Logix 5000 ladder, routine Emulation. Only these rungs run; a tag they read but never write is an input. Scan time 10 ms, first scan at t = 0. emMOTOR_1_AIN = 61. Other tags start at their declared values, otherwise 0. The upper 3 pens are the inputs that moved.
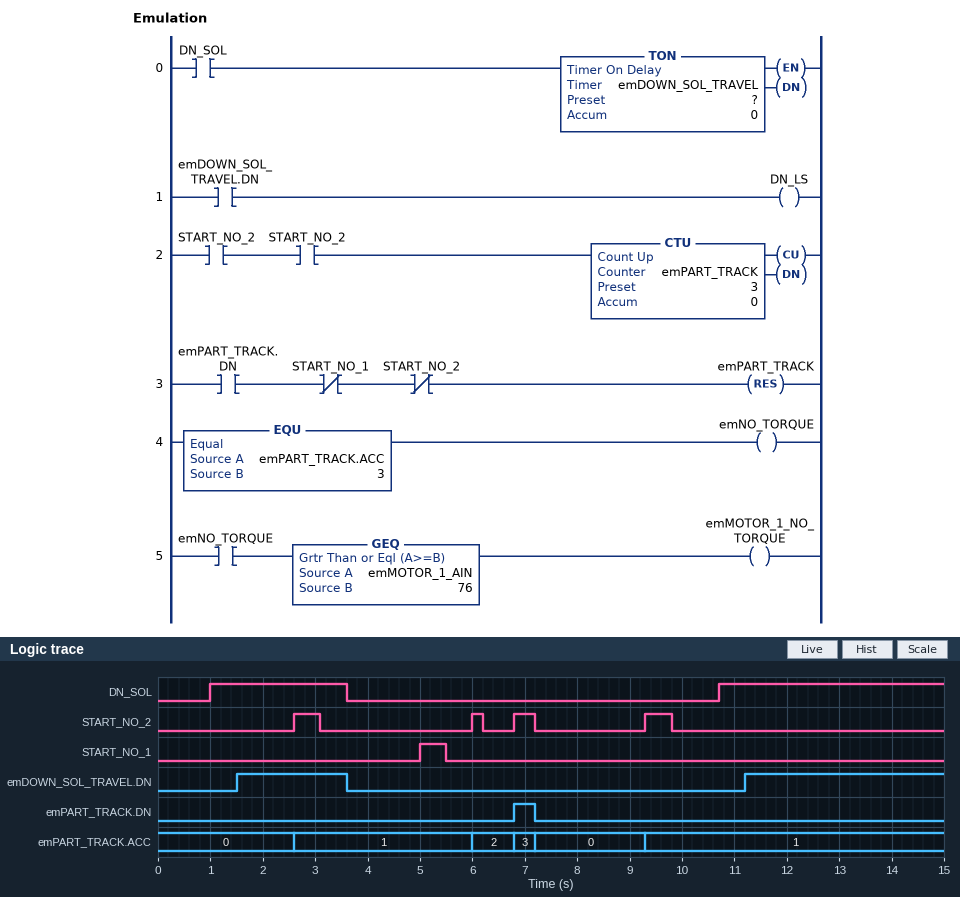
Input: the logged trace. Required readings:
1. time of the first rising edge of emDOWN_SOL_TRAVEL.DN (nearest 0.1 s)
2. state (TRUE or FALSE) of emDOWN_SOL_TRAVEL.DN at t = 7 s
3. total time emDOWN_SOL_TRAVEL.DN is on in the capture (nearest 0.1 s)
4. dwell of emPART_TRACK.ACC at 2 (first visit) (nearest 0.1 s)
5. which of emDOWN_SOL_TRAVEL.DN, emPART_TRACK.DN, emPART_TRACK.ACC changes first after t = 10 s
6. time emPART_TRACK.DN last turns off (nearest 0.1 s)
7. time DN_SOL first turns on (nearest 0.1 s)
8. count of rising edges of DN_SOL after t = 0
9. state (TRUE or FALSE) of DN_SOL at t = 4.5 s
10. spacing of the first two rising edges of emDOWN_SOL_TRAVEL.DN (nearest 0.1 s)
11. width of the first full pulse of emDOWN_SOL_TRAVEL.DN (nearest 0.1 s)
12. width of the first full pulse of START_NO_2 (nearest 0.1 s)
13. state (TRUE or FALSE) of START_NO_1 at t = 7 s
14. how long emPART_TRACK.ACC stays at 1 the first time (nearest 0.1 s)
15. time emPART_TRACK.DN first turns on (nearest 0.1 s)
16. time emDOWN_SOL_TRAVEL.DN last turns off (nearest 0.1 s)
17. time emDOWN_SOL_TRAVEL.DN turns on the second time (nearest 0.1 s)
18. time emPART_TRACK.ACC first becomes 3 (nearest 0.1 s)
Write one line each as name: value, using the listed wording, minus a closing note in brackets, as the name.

time of the first rising edge of emDOWN_SOL_TRAVEL.DN: 1.5 s
state (TRUE or FALSE) of emDOWN_SOL_TRAVEL.DN at t = 7 s: FALSE
total time emDOWN_SOL_TRAVEL.DN is on in the capture: 5.9 s
dwell of emPART_TRACK.ACC at 2 (first visit): 0.8 s
which of emDOWN_SOL_TRAVEL.DN, emPART_TRACK.DN, emPART_TRACK.ACC changes first after t = 10 s: emDOWN_SOL_TRAVEL.DN
time emPART_TRACK.DN last turns off: 7.2 s
time DN_SOL first turns on: 1.0 s
count of rising edges of DN_SOL after t = 0: 2
state (TRUE or FALSE) of DN_SOL at t = 4.5 s: FALSE
spacing of the first two rising edges of emDOWN_SOL_TRAVEL.DN: 9.7 s
width of the first full pulse of emDOWN_SOL_TRAVEL.DN: 2.1 s
width of the first full pulse of START_NO_2: 0.5 s
state (TRUE or FALSE) of START_NO_1 at t = 7 s: FALSE
how long emPART_TRACK.ACC stays at 1 the first time: 3.4 s
time emPART_TRACK.DN first turns on: 6.8 s
time emDOWN_SOL_TRAVEL.DN last turns off: 3.6 s
time emDOWN_SOL_TRAVEL.DN turns on the second time: 11.2 s
time emPART_TRACK.ACC first becomes 3: 6.8 s
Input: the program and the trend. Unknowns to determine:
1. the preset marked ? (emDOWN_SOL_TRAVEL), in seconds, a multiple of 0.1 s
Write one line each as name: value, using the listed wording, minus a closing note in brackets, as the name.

the preset marked ? (emDOWN_SOL_TRAVEL), in seconds, a multiple of 0.1 s: 0.5 s
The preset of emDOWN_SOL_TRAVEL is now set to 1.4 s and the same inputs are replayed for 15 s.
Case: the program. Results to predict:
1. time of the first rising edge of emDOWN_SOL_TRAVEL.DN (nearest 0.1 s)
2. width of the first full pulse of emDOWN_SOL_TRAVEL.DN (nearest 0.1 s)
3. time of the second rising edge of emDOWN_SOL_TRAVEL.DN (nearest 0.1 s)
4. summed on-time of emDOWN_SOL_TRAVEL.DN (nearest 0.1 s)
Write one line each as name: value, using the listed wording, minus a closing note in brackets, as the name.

time of the first rising edge of emDOWN_SOL_TRAVEL.DN: 2.4 s
width of the first full pulse of emDOWN_SOL_TRAVEL.DN: 1.2 s
time of the second rising edge of emDOWN_SOL_TRAVEL.DN: 12.1 s
summed on-time of emDOWN_SOL_TRAVEL.DN: 4.1 s
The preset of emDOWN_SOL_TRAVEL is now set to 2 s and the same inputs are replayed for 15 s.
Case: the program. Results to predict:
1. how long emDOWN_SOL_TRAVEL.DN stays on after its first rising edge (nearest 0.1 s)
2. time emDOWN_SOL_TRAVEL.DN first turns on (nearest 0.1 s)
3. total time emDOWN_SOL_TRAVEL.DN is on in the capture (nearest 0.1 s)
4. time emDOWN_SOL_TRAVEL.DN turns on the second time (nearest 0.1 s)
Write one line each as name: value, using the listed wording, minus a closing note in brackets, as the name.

how long emDOWN_SOL_TRAVEL.DN stays on after its first rising edge: 0.6 s
time emDOWN_SOL_TRAVEL.DN first turns on: 3.0 s
total time emDOWN_SOL_TRAVEL.DN is on in the capture: 2.9 s
time emDOWN_SOL_TRAVEL.DN turns on the second time: 12.7 s
